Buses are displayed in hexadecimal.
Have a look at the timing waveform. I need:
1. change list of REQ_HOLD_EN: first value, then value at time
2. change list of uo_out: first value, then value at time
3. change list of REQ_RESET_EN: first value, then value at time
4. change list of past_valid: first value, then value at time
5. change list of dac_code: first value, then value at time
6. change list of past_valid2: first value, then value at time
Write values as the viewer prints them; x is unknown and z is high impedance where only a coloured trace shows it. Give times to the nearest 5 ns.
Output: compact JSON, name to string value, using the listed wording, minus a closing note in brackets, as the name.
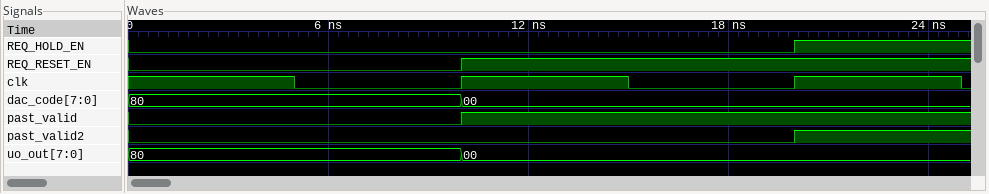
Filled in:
{"change list of REQ_HOLD_EN: first value, then value at time": "0, 1 at 20 ns", "change list of uo_out: first value, then value at time": "80, 00 at 10 ns", "change list of REQ_RESET_EN: first value, then value at time": "0, 1 at 10 ns", "change list of past_valid: first value, then value at time": "0, 1 at 10 ns", "change list of dac_code: first value, then value at time": "80, 00 at 10 ns", "change list of past_valid2: first value, then value at time": "0, 1 at 20 ns"}
